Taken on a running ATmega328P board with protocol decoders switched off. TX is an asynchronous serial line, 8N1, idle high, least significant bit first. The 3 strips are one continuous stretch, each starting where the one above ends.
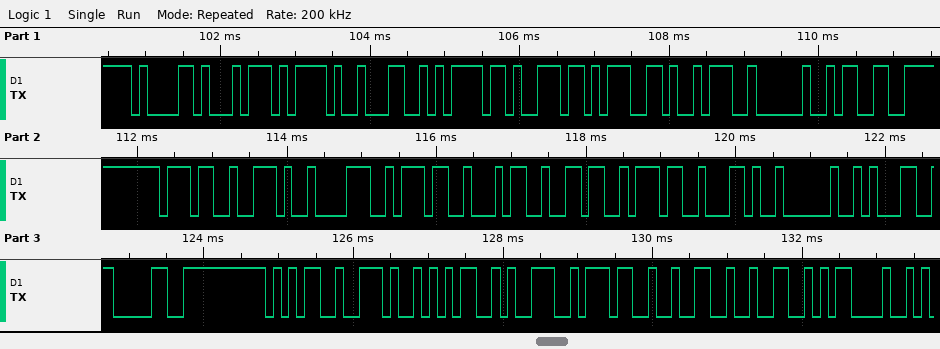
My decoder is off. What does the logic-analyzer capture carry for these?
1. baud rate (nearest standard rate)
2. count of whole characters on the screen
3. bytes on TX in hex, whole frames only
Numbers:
9600 baud
29
61 74 2F 4C 6F 6E 67 3A 20 33 37 2E 38 37 34 36 37 2C 20 31 30 35 2E 35 39 37 32 32 0D
